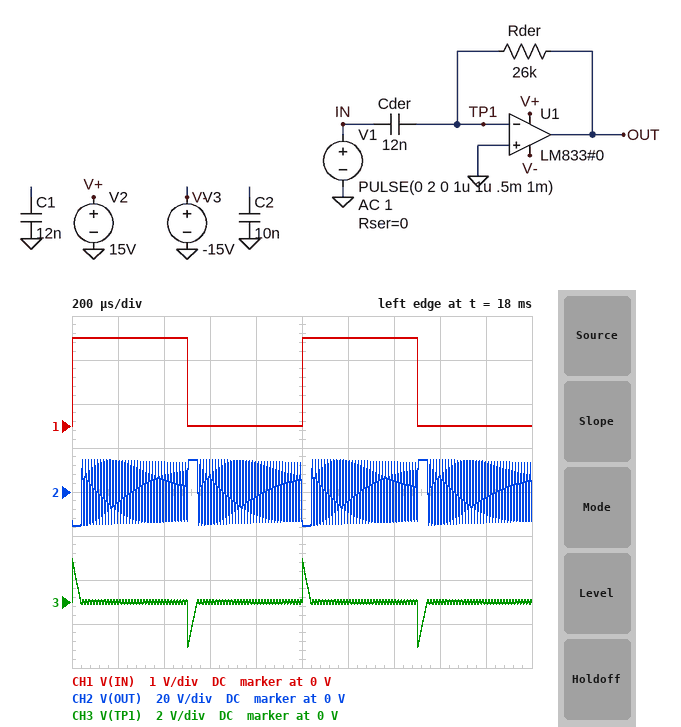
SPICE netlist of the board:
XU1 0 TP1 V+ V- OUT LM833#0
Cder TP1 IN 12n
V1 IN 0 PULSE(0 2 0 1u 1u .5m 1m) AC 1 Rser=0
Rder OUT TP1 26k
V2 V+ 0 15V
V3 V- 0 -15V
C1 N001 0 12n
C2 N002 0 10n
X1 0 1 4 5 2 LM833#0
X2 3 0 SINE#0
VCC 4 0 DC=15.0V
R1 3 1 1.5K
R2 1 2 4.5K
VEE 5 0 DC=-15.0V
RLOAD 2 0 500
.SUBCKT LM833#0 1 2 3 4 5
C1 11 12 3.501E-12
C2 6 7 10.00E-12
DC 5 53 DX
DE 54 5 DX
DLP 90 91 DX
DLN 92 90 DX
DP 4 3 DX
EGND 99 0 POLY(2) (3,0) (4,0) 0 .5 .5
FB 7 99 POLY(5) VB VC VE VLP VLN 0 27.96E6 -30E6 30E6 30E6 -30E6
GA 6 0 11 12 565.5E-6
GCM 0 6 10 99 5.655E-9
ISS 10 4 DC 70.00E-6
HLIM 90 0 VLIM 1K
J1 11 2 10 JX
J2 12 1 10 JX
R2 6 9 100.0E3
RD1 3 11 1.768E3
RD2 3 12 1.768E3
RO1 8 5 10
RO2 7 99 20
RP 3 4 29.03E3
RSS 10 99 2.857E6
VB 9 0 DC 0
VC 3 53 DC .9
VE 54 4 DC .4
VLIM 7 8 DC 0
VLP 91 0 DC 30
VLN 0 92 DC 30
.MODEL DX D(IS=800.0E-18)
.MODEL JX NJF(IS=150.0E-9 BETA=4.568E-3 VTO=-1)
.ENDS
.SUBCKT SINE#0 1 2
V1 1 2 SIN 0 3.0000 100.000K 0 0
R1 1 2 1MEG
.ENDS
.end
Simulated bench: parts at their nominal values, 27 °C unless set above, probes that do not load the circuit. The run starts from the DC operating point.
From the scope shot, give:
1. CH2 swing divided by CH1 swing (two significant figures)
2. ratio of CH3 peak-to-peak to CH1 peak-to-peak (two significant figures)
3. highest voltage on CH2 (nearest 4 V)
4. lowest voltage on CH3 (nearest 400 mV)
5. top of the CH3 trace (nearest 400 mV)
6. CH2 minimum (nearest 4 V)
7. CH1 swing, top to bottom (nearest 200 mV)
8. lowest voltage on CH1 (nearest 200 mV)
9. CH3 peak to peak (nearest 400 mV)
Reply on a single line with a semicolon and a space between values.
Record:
15; 2.0; 16 V; -2.0 V; 2.0 V; -16 V; 2.0 V; 0 V; 4.0 V
